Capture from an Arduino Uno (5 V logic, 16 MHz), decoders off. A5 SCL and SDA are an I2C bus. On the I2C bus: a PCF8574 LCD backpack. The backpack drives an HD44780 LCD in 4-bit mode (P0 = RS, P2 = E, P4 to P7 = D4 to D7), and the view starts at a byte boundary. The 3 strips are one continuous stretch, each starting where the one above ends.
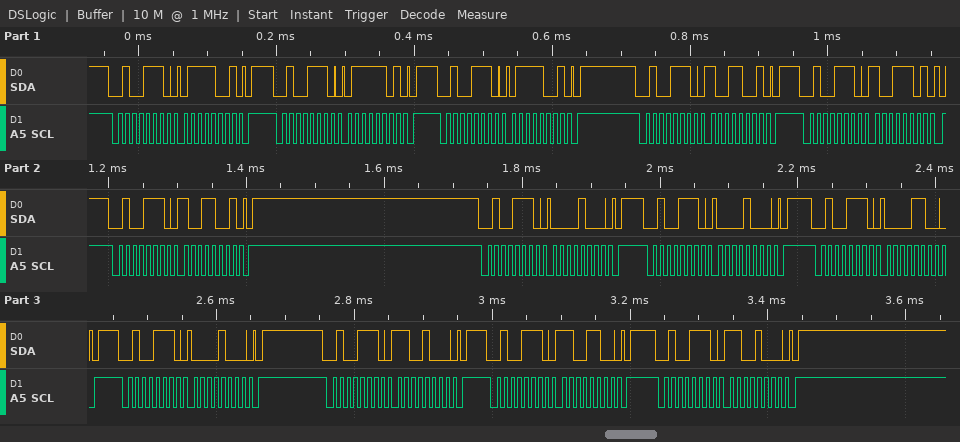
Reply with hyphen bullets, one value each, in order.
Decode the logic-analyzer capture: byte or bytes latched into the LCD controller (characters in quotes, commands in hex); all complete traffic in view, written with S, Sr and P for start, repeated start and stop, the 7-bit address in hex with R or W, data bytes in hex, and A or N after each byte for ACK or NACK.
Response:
- 'y' 0x0C
- S 27W A 79 A P S 27W A 7D A P S 27W A 79 A P S 27W A 99 A P S 27W A 9D A P S 27W A 99 A P S 27W A 08 A P S 27W A 08 A P S 27W A 0C A P S 27W A 08 A P S 27W A C8 A P S 27W A CC A P S 27W A C8 A P
